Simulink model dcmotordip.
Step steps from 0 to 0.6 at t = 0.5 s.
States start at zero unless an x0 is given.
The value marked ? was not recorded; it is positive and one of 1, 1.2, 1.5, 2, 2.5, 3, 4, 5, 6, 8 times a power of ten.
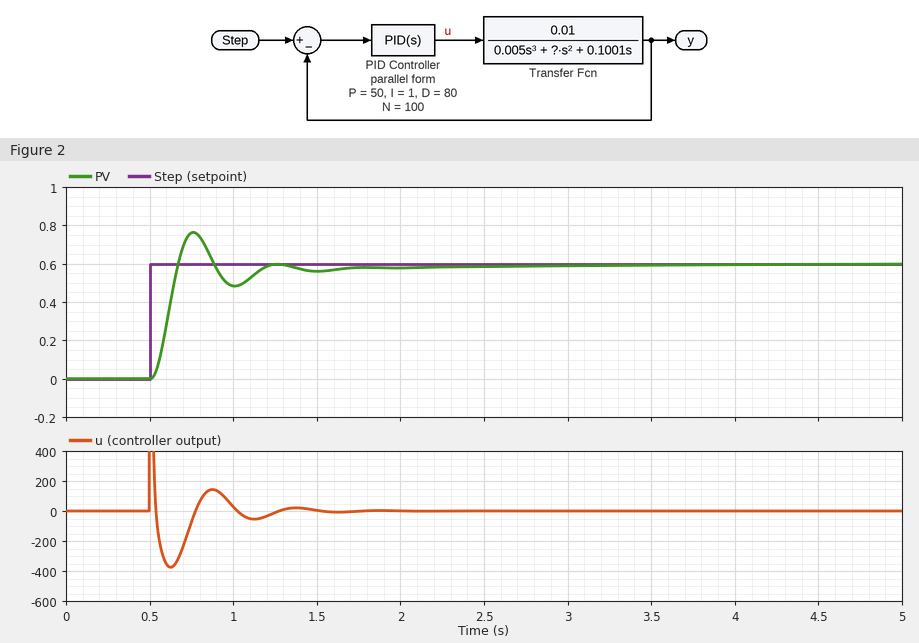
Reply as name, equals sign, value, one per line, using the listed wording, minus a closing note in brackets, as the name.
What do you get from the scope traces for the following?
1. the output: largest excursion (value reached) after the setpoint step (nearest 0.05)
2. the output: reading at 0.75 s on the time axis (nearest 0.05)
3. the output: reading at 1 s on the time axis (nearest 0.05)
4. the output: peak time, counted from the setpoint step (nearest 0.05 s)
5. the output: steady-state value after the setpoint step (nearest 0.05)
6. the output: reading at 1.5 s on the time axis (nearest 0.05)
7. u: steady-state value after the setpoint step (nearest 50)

the output: largest excursion (value reached) after the setpoint step = 0.75
the output: reading at 0.75 s on the time axis = 0.75
the output: reading at 1 s on the time axis = 0.50
the output: peak time, counted from the setpoint step = 0.25 s
the output: steady-state value after the setpoint step = 0.60
the output: reading at 1.5 s on the time axis = 0.55
u: steady-state value after the setpoint step = 0
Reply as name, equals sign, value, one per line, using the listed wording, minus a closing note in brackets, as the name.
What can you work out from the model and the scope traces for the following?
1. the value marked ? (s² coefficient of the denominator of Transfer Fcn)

the value marked ? = 0.05
